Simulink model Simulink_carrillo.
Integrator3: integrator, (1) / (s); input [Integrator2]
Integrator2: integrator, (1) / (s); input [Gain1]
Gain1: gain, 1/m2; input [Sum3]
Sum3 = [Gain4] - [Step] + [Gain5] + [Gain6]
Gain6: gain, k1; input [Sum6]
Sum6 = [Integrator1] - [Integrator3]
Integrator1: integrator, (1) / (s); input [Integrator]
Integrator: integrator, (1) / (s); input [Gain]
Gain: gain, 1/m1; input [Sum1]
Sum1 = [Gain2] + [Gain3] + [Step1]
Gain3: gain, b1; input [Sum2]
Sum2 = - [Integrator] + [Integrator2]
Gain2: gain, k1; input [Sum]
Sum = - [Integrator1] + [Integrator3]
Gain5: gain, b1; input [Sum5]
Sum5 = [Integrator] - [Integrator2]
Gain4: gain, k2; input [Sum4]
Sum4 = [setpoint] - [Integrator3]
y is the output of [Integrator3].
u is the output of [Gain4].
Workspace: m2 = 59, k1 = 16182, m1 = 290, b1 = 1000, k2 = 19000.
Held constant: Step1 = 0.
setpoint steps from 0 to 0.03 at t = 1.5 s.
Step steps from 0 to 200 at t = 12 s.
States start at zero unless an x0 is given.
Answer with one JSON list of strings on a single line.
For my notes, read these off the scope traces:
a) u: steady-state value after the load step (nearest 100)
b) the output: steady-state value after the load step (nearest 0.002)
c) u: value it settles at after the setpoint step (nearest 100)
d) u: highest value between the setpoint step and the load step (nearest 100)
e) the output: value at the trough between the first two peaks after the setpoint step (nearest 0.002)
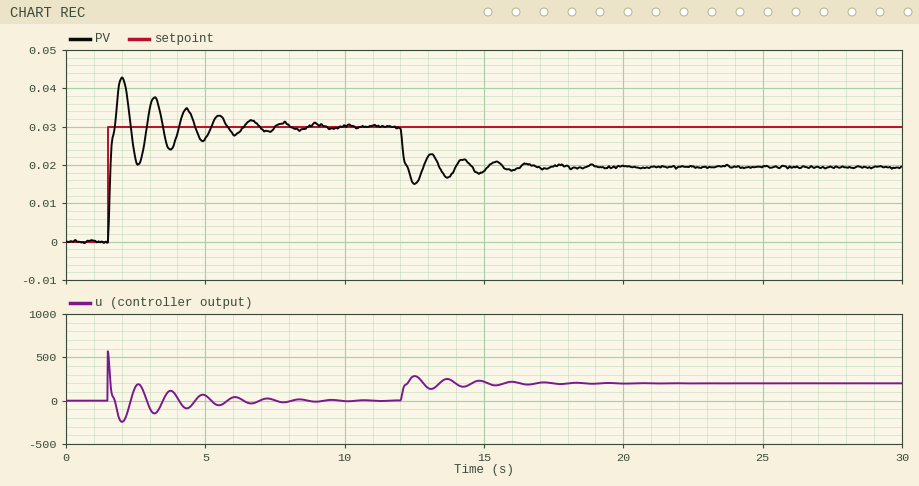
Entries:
["200", "0.020", "0", "600", "0.020"]
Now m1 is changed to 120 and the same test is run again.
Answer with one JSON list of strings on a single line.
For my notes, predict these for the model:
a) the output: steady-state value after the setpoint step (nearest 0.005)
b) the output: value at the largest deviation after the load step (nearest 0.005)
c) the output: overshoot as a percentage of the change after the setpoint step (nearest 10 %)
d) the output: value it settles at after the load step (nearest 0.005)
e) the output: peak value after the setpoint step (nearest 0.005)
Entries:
["0.030", "0.015", "50 %", "0.020", "0.045"]
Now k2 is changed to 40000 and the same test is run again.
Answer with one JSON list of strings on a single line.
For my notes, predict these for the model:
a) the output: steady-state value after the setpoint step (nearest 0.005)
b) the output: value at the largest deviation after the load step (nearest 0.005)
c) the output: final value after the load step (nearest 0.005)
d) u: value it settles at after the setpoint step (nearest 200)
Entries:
["0.030", "0.025", "0.025", "0"]
